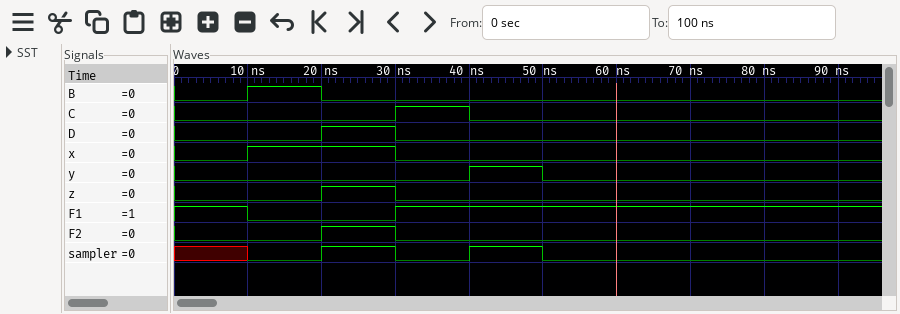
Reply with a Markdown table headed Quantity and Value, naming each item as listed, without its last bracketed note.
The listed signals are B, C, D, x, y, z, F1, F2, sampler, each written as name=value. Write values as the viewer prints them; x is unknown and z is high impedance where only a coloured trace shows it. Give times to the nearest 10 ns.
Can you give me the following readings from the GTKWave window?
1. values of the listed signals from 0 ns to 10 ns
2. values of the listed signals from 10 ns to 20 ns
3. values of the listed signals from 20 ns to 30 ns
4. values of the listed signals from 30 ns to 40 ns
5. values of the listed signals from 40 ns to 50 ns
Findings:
| Quantity | Value |
|---|---|
| values of the listed signals from 0 ns to 10 ns | B=0, C=0, D=0, x=0, y=0, z=0, F1=1, F2=0, sampler=x |
| values of the listed signals from 10 ns to 20 ns | B=1, C=0, D=0, x=1, y=0, z=0, F1=0, F2=0, sampler=0 |
| values of the listed signals from 20 ns to 30 ns | B=0, C=0, D=1, x=1, y=0, z=1, F1=0, F2=1, sampler=1 |
| values of the listed signals from 30 ns to 40 ns | B=0, C=1, D=0, x=0, y=0, z=0, F1=1, F2=0, sampler=0 |
| values of the listed signals from 40 ns to 50 ns | B=0, C=0, D=0, x=0, y=1, z=0, F1=1, F2=0, sampler=1 |
